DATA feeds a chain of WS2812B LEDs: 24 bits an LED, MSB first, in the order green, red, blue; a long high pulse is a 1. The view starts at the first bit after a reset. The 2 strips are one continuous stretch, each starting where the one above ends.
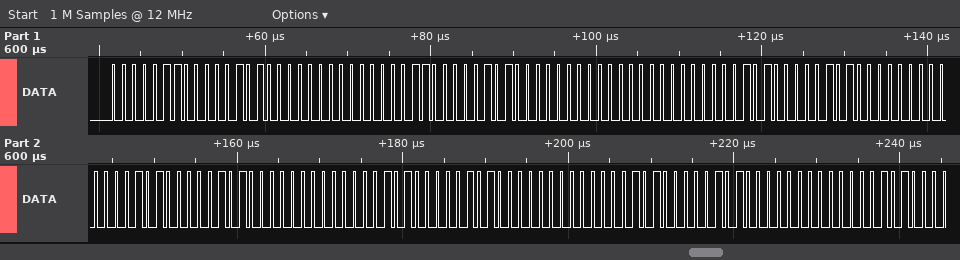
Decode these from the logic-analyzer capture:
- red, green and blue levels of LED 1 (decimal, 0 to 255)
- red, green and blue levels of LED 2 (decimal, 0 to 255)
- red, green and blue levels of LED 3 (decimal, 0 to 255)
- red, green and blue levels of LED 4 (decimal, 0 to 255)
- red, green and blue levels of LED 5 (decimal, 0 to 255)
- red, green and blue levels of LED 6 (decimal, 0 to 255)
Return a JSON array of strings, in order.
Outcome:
["10, 6, 0", "10, 6, 0", "5, 0, 5", "5, 0, 5", "5, 0, 5", "5, 0, 5"]
